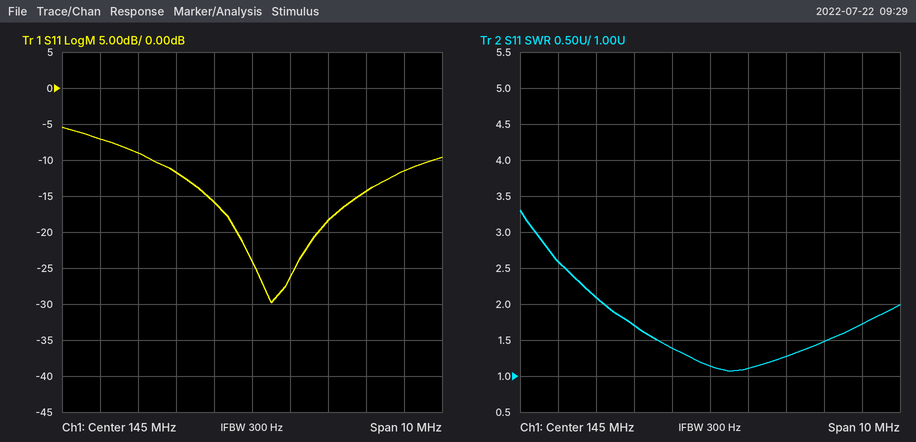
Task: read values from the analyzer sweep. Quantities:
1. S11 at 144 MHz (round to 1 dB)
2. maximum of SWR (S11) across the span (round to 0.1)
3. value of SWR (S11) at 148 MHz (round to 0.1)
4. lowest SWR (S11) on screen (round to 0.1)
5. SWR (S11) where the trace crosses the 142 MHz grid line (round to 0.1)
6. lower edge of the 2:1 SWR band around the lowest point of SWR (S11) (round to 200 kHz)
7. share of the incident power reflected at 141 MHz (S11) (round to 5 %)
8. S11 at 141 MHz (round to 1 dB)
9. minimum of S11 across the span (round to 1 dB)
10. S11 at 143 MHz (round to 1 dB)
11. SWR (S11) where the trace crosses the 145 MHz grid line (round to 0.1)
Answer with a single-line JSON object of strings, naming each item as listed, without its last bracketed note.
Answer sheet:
{"S11 at 144 MHz": "-16 dB", "maximum of SWR (S11) across the span": "3.3", "value of SWR (S11) at 148 MHz": "1.5", "lowest SWR (S11) on screen": "1.1", "SWR (S11) where the trace crosses the 142 MHz grid line": "2.1", "lower edge of the 2:1 SWR band around the lowest point of SWR (S11)": "142.2 MHz", "share of the incident power reflected at 141 MHz (S11)": "20 %", "S11 at 141 MHz": "-7 dB", "minimum of S11 across the span": "-30 dB", "S11 at 143 MHz": "-12 dB", "SWR (S11) where the trace crosses the 145 MHz grid line": "1.1"}
